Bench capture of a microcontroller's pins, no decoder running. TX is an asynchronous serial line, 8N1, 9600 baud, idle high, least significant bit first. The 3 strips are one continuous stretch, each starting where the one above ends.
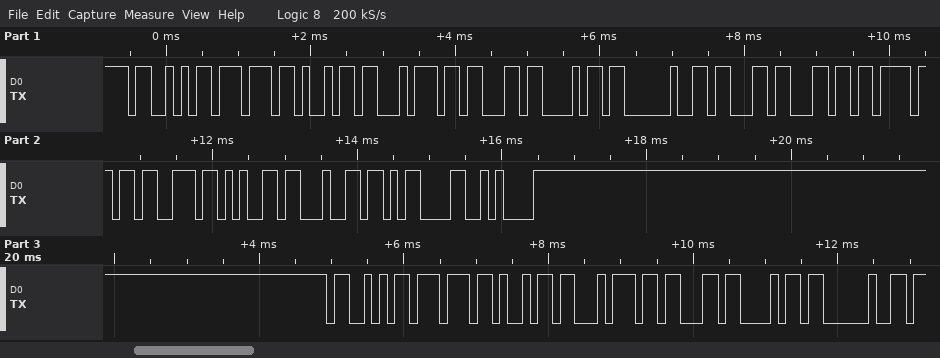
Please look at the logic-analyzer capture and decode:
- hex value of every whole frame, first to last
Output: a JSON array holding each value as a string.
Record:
["0x53 0x77 0x69 0x74 0x63 0x68 0x20 0x63 0x6C 0x6F 0x73 0x65 0x64 0x0D 0x0A 0x53 0x77 0x69 0x74 0x63 0x68 0x20"]
